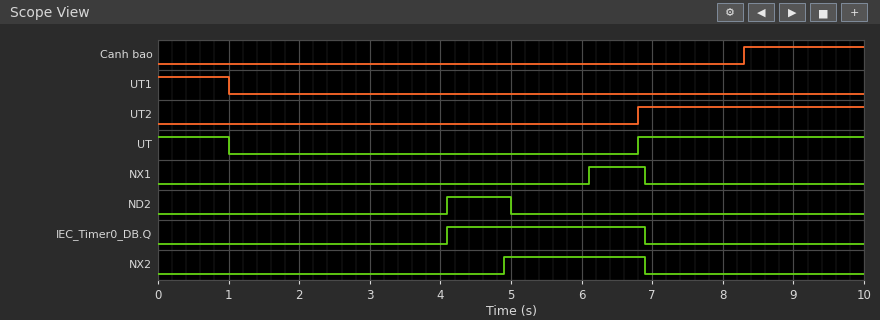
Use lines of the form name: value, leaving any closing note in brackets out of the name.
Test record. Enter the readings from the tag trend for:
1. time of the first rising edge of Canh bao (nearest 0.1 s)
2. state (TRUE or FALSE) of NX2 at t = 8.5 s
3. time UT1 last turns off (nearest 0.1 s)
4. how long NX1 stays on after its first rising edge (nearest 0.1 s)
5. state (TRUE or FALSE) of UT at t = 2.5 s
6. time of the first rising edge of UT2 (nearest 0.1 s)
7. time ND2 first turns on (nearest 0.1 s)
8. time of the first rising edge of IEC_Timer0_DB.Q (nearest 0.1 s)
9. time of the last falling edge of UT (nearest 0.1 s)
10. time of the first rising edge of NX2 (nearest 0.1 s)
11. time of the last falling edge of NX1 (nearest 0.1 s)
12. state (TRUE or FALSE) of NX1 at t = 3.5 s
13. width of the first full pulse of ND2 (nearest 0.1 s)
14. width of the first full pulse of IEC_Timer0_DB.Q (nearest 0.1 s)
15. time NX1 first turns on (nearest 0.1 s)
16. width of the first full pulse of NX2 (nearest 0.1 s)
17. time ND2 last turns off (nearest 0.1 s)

time of the first rising edge of Canh bao: 8.3 s
state (TRUE or FALSE) of NX2 at t = 8.5 s: FALSE
time UT1 last turns off: 1.0 s
how long NX1 stays on after its first rising edge: 0.8 s
state (TRUE or FALSE) of UT at t = 2.5 s: FALSE
time of the first rising edge of UT2: 6.8 s
time ND2 first turns on: 4.1 s
time of the first rising edge of IEC_Timer0_DB.Q: 4.1 s
time of the last falling edge of UT: 1.0 s
time of the first rising edge of NX2: 4.9 s
time of the last falling edge of NX1: 6.9 s
state (TRUE or FALSE) of NX1 at t = 3.5 s: FALSE
width of the first full pulse of ND2: 0.9 s
width of the first full pulse of IEC_Timer0_DB.Q: 2.8 s
time NX1 first turns on: 6.1 s
width of the first full pulse of NX2: 2.0 s
time ND2 last turns off: 5.0 s
